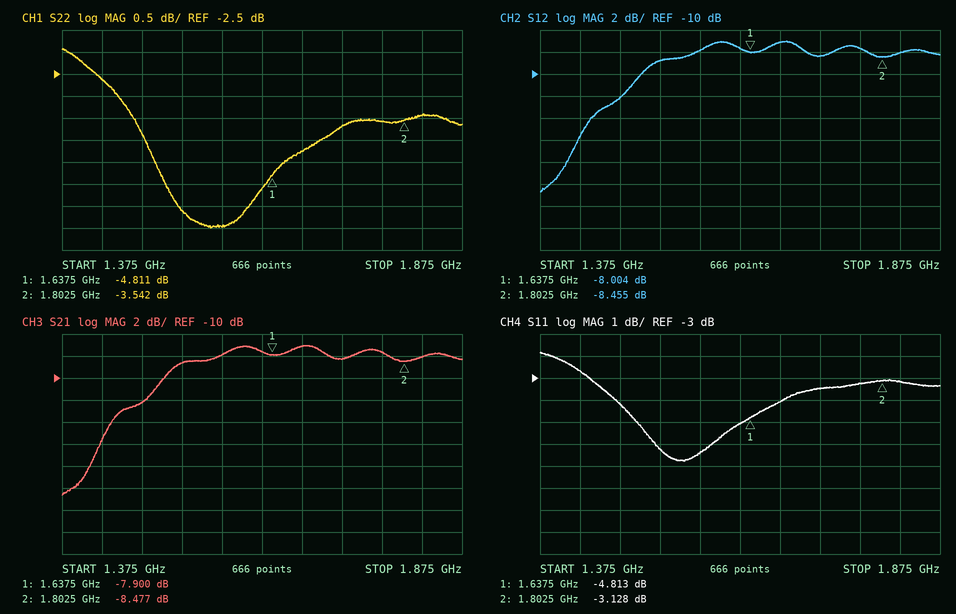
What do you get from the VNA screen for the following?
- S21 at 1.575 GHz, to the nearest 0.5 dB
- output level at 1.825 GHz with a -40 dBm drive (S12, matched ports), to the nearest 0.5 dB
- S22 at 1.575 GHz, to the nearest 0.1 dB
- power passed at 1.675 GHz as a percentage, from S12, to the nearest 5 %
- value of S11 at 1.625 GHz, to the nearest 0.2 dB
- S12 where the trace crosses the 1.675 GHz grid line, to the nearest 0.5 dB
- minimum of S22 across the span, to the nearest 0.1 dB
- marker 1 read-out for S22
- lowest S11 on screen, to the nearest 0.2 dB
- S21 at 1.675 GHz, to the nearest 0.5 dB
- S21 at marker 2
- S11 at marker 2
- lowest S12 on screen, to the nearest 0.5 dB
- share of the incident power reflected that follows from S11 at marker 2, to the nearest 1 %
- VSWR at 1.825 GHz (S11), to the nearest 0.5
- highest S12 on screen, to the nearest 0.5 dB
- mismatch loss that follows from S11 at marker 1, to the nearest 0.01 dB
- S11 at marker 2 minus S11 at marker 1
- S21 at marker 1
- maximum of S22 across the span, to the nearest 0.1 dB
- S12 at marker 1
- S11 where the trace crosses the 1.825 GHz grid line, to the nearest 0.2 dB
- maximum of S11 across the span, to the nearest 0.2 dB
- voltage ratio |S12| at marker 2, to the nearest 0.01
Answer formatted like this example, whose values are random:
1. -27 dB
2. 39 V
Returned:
1. -8.0 dB
2. -48.0 dBm
3. -6.0 dB
4. 20 %
5. -5.0 dB
6. -7.0 dB
7. -6.0 dB
8. -4.811 dB
9. -6.8 dB
10. -7.0 dB
11. -8.477 dB
12. -3.128 dB
13. -20.5 dB
14. 49 %
15. 5.5
16. -7.0 dB
17. 1.74 dB
18. 1.685 dB
19. -7.900 dB
20. -1.9 dB
21. -8.004 dB
22. -3.2 dB
23. -1.8 dB
24. 0.38
